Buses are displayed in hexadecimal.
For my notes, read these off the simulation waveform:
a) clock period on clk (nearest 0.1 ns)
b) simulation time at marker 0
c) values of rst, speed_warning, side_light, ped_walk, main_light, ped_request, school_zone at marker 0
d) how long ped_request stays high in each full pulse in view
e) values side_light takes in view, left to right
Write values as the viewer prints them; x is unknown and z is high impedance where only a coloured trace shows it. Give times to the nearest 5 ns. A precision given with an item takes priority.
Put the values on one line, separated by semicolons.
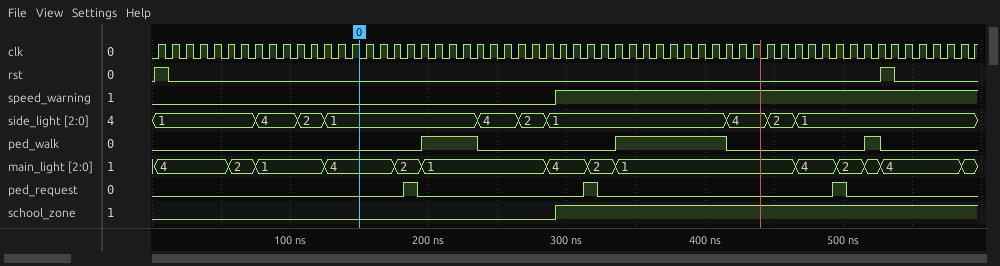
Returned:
10 ns; 150 ns; rst=0, speed_warning=0, side_light=1, ped_walk=0, main_light=4, ped_request=0, school_zone=0; 10 ns, 10 ns, 10 ns; 1, 4, 2, 1, 4, 2, 1, 4, 2, 1
